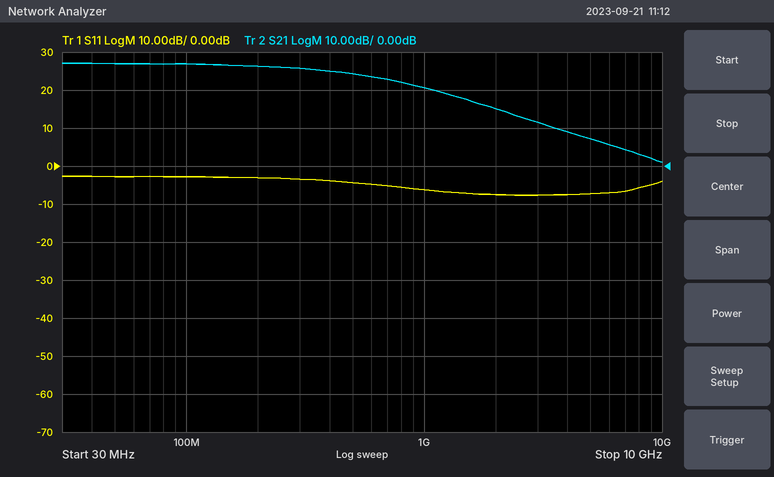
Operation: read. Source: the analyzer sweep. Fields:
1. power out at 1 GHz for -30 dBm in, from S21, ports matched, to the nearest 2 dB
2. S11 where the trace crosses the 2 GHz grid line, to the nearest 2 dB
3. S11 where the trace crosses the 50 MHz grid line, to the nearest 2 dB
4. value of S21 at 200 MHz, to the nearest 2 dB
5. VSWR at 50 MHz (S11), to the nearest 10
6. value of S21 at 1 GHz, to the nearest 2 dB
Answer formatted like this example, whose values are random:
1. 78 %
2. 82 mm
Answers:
1. -10 dBm
2. -8 dB
3. -2 dB
4. 26 dB
5. 10
6. 20 dB
